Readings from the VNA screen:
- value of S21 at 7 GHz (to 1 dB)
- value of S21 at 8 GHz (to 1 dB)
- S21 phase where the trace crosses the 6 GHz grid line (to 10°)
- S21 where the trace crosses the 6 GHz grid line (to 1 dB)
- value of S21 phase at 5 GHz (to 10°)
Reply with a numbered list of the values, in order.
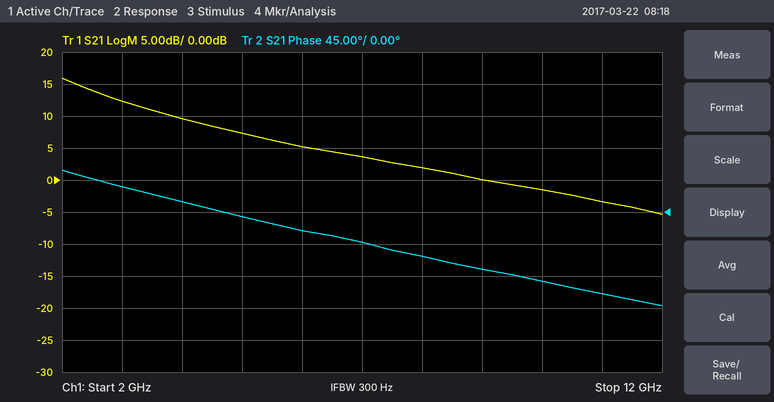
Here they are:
1. 4 dB
2. 2 dB
3. -30°
4. 5 dB
5. -10°
